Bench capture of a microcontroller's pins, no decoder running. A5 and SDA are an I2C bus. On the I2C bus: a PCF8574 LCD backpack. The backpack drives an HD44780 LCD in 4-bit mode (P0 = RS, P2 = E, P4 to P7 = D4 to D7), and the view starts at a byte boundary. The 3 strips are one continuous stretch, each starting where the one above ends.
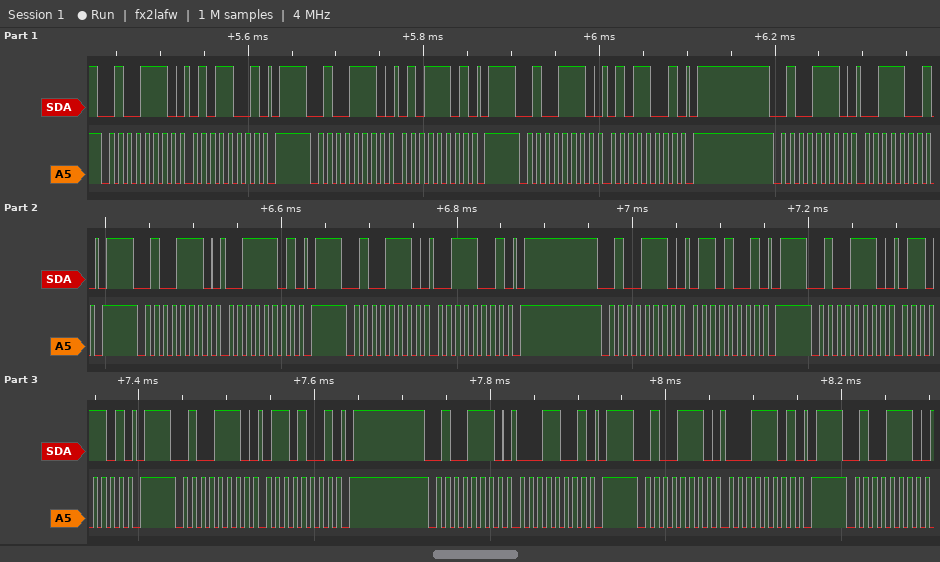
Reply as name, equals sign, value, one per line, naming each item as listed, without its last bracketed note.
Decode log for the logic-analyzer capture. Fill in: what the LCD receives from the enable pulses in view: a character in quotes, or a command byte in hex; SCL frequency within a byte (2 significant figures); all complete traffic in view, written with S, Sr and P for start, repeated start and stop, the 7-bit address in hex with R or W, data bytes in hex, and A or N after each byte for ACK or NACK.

what the LCD receives from the enable pulses in view: a character in quotes, or a command byte in hex = 'S'
SCL frequency within a byte = 100 kHz
all complete traffic in view, written with S, Sr and P for start, repeated start and stop, the 7-bit address in hex with R or W, data bytes in hex, and A or N after each byte for ACK or NACK = S 27W A 59 A P S 27W A 5D A P S 27W A 59 A P S 27W A 39 A P S 27W A 3D A P S 27W A 39 A P S 27W A 69 A P S 27W A 6D A P S 27W A 69 A P S 27W A 19 A P S 27W A 1D A P S 27W A
